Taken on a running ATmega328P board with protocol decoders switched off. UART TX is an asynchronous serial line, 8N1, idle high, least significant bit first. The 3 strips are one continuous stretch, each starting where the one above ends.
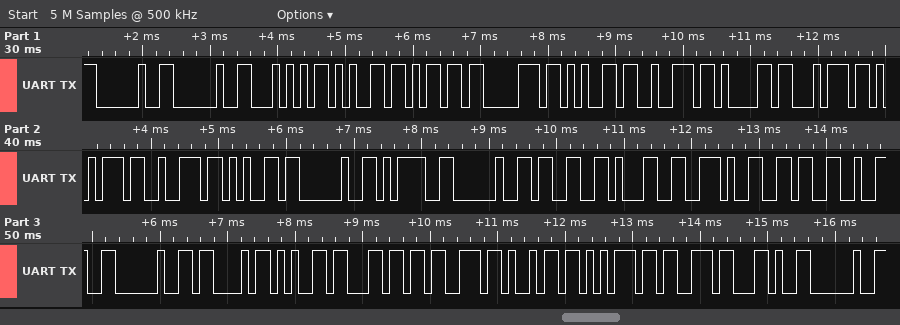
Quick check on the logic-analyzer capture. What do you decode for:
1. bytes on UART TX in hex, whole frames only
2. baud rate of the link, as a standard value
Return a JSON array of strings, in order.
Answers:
["20 20 54 65 6D 70 65 72 61 74 75 72 65 20 3D 20 33 31 2E 36 32 20 43 65 6C 73 69 75 73 2C 20", "9600 baud"]
